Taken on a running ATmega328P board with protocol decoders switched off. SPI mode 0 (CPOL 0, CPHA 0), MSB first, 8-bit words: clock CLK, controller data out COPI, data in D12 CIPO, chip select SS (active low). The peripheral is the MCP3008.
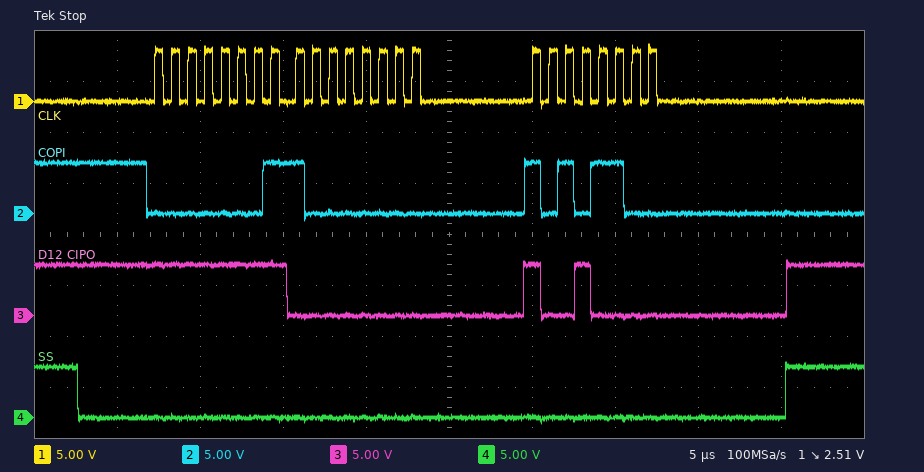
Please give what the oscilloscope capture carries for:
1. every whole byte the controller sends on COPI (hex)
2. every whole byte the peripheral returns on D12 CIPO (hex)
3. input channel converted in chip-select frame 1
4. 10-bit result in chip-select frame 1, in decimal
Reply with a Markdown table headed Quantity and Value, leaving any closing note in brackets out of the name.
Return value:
| Quantity | Value |
|---|---|
| every whole byte the controller sends on COPI | 01 80 AC |
| every whole byte the peripheral returns on D12 CIPO | FF 00 90 |
| input channel converted in chip-select frame 1 | 0 |
| 10-bit result in chip-select frame 1, in decimal | 144 |
